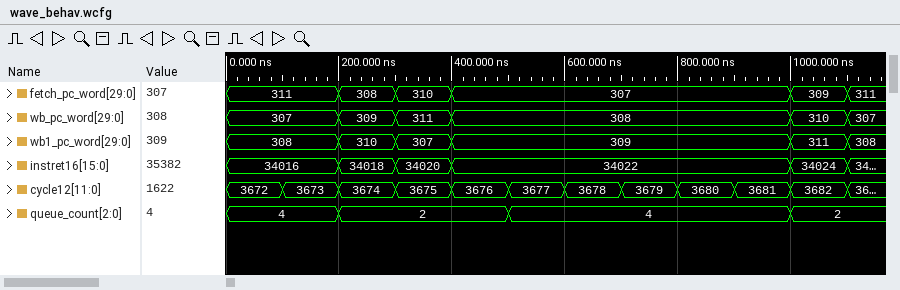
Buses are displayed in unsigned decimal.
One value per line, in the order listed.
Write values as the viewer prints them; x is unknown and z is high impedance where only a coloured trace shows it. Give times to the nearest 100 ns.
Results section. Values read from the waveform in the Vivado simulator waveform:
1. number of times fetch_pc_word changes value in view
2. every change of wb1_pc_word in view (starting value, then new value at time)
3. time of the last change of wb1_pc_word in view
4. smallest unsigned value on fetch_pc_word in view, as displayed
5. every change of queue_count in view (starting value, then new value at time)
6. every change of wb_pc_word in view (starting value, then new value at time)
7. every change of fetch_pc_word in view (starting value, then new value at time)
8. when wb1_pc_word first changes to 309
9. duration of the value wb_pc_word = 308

5
308, 310 at 200 ns, 307 at 300 ns, 309 at 400 ns, 311 at 1000 ns, 308 at 1100 ns
1100 ns
307
4, 2 at 200 ns, 4 at 500 ns, 2 at 1000 ns
307, 309 at 200 ns, 311 at 300 ns, 308 at 400 ns, 310 at 1000 ns, 307 at 1100 ns
311, 308 at 200 ns, 310 at 300 ns, 307 at 400 ns, 309 at 1000 ns, 311 at 1100 ns
400 ns
600 ns
